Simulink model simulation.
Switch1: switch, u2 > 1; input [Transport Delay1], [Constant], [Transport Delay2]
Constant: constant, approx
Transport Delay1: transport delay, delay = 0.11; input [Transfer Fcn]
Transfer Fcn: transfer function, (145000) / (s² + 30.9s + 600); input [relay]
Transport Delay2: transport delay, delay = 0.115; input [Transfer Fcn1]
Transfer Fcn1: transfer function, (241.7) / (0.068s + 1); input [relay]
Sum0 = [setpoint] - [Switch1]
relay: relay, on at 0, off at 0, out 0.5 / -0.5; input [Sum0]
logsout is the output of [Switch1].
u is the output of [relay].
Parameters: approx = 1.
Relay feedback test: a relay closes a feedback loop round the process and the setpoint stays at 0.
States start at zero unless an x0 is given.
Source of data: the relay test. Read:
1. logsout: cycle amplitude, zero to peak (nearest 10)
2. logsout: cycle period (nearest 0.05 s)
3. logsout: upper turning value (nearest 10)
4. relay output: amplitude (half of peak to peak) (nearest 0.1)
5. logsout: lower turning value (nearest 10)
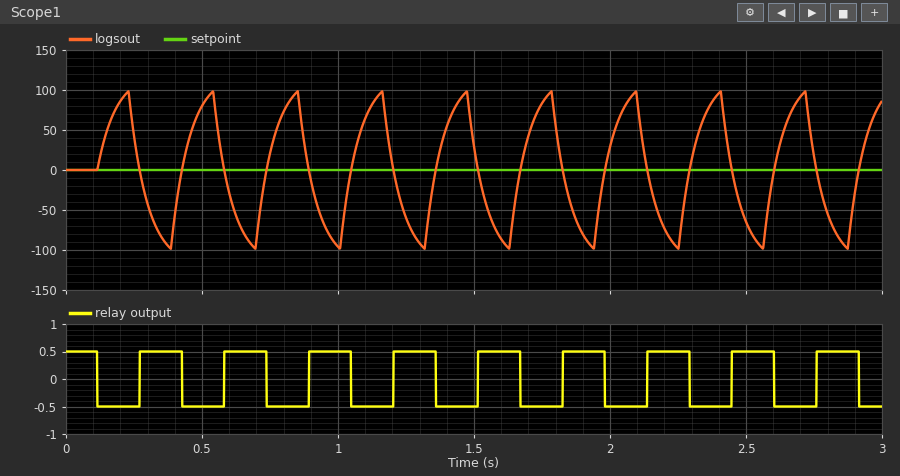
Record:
100
0.30 s
100
0.5
-100
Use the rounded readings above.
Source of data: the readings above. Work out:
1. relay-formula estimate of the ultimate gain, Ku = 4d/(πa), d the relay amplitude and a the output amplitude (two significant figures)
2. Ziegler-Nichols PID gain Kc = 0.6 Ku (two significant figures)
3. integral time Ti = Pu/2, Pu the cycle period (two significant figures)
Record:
0.0064
0.0038
0.15 s
